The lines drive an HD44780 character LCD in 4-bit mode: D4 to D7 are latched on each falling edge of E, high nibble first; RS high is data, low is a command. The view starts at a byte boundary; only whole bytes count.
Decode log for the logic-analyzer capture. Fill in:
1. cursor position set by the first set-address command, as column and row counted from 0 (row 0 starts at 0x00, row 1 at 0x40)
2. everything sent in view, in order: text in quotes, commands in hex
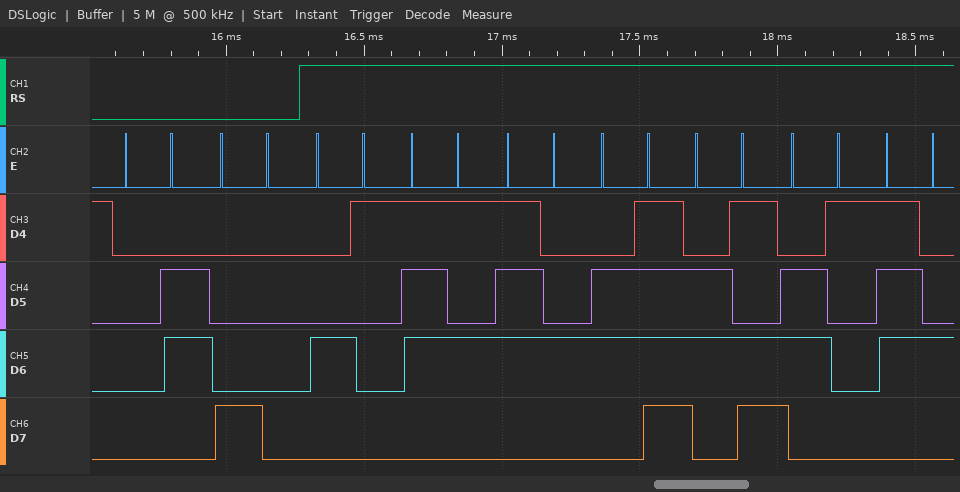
column 0, row 0
0x06 0x80 "Automat"
